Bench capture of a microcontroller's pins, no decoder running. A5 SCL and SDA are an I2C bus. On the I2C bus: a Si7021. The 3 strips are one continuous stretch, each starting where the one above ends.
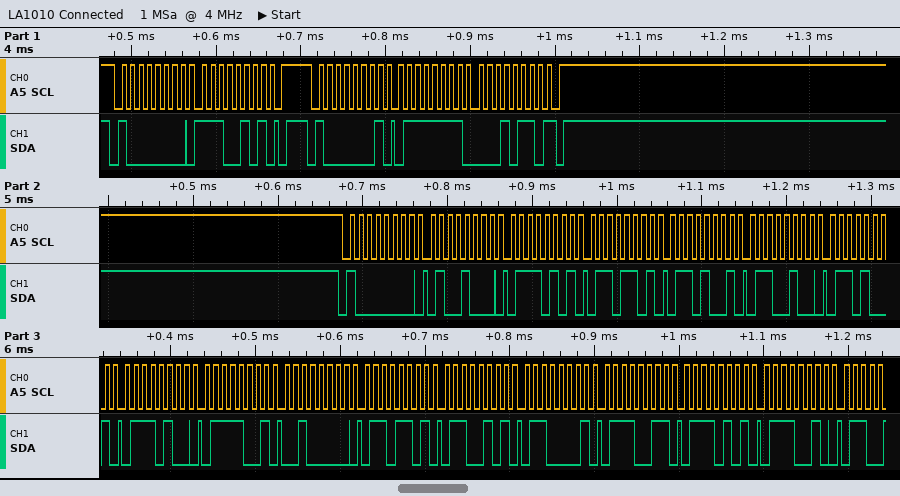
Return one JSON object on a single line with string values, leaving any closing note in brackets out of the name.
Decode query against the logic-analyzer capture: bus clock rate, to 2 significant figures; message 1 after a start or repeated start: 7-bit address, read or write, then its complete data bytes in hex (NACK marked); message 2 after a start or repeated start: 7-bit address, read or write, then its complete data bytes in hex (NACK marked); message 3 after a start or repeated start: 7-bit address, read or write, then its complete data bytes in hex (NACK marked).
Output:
{"bus clock rate, to 2 significant figures": "100 kHz", "message 1 after a start or repeated start: 7-bit address, read or write, then its complete data bytes in hex": "0x40 write: E5", "message 2 after a start or repeated start: 7-bit address, read or write, then its complete data bytes in hex": "0x40 read: 7F 16 NACK", "message 3 after a start or repeated start: 7-bit address, read or write, then its complete data bytes in hex": "0x40 write: 48 75 6D 69 64 69 74 79 20 6D 65 61 73 75 72"}
